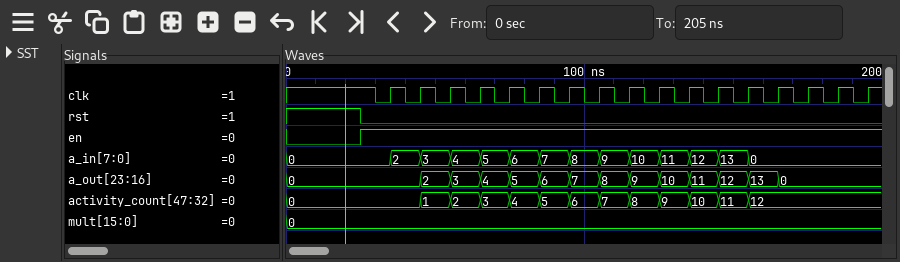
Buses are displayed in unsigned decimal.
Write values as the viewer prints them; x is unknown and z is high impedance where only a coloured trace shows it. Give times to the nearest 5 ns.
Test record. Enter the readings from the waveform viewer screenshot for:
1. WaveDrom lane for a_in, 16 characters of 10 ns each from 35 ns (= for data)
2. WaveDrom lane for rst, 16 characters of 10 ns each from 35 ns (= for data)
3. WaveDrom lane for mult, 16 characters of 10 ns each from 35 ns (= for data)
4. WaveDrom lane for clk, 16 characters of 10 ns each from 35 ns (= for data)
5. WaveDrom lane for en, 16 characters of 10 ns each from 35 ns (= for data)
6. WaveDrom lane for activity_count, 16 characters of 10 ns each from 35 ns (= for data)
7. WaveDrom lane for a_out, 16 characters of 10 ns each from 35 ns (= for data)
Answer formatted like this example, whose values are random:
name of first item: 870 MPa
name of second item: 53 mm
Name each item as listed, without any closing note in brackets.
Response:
WaveDrom lane for a_in, 16 characters of 10 ns each from 35 ns: {name: 'a_in', wave: '=============...', data: '2 3 4 5 6 7 8 9 10 11 12 13 0'}
WaveDrom lane for rst, 16 characters of 10 ns each from 35 ns: {name: 'rst', wave: '0...............'}
WaveDrom lane for mult, 16 characters of 10 ns each from 35 ns: {name: 'mult', wave: '=...............', data: '0'}
WaveDrom lane for clk, 16 characters of 10 ns each from 35 ns: {name: 'clk', wave: 'p...............'}
WaveDrom lane for en, 16 characters of 10 ns each from 35 ns: {name: 'en', wave: '1...............'}
WaveDrom lane for activity_count, 16 characters of 10 ns each from 35 ns: {name: 'activity_count', wave: '=============...', data: '0 1 2 3 4 5 6 7 8 9 10 11 12'}
WaveDrom lane for a_out, 16 characters of 10 ns each from 35 ns: {name: 'a_out', wave: '==============..', data: '0 2 3 4 5 6 7 8 9 10 11 12 13 0'}
